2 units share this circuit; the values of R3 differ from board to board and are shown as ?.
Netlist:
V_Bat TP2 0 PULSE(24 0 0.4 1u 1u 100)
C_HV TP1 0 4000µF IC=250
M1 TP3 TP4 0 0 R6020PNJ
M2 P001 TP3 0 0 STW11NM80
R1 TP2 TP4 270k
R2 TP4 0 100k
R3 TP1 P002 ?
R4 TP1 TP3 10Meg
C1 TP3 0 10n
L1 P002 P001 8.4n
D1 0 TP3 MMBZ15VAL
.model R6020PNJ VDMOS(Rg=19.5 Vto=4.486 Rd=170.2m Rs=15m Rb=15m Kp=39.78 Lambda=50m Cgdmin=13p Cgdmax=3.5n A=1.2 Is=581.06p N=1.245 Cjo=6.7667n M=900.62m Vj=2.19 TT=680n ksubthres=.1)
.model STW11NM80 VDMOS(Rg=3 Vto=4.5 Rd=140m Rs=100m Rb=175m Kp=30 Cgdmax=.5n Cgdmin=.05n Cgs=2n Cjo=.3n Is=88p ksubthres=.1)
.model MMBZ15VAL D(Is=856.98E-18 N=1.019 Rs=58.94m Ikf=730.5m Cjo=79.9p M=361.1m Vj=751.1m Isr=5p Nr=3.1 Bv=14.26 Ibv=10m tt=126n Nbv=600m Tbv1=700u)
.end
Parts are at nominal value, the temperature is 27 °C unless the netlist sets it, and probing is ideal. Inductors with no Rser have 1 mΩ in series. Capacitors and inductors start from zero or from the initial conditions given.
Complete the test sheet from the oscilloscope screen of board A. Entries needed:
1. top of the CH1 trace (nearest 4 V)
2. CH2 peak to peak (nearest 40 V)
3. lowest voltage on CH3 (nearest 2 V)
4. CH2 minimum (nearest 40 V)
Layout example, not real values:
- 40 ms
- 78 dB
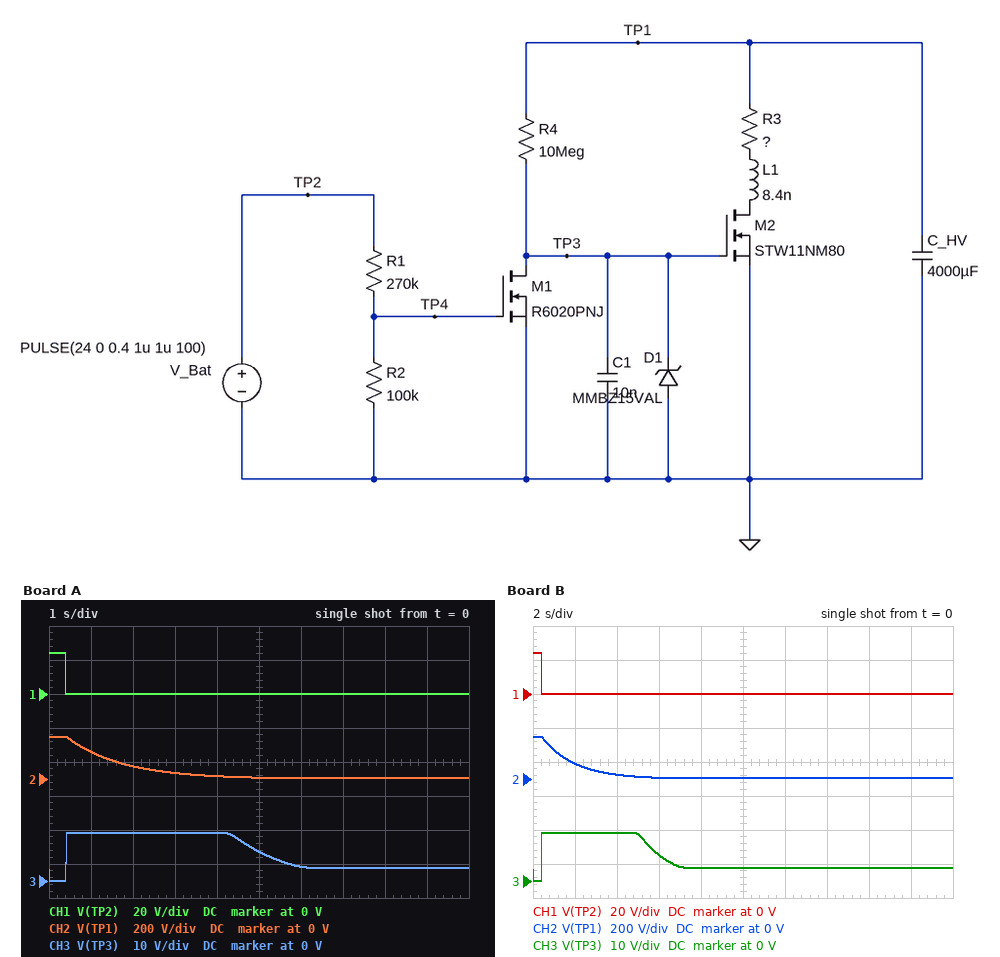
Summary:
- 24 V
- 240 V
- 0 V
- 0 V
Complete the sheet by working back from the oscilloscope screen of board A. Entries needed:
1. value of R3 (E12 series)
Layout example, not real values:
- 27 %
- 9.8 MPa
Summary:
- 330 Ω
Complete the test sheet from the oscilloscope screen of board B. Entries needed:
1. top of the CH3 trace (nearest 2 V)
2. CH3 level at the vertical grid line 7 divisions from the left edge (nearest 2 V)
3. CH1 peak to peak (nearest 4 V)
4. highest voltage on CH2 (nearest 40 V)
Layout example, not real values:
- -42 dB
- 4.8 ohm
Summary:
- 14 V
- 4 V
- 24 V
- 240 V
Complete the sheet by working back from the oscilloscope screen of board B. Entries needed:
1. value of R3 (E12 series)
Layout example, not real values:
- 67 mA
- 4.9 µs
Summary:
- 390 Ω
